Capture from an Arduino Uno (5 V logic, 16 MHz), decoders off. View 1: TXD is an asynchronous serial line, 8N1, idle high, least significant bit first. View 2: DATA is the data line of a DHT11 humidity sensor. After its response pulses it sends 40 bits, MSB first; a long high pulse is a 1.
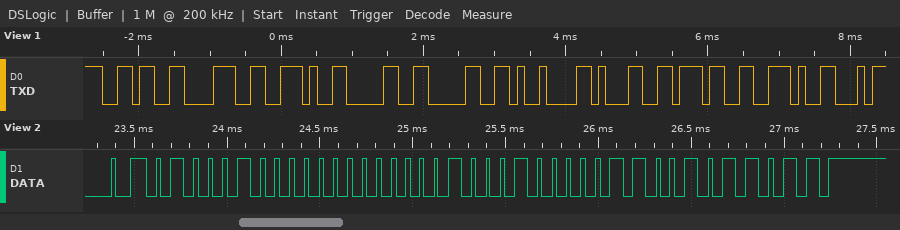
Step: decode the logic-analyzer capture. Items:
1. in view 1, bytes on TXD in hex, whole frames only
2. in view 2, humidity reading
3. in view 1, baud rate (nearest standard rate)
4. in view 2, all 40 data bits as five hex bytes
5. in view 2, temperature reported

36 38 2E 30 30 09 31 37 2E
68 %
9600 baud
44 00 11 06 5B
17.6 °C
